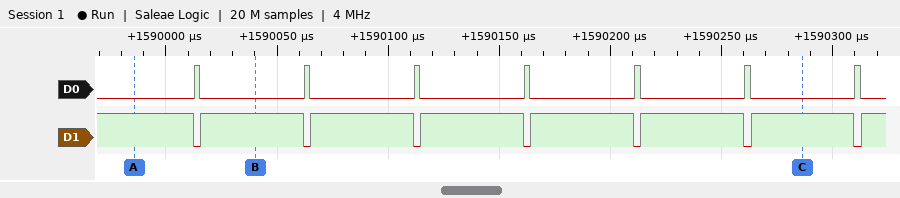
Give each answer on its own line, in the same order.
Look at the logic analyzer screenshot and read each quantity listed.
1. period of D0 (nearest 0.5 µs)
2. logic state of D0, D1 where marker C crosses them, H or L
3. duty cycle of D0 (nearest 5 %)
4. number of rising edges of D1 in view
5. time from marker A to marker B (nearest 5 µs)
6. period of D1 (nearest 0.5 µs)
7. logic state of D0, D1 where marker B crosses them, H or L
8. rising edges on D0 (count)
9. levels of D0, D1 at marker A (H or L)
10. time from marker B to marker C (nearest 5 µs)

49.5 µs
D0=L, D1=H
5 %
7
55 µs
49.5 µs
D0=L, D1=H
7
D0=L, D1=H
245 µs
